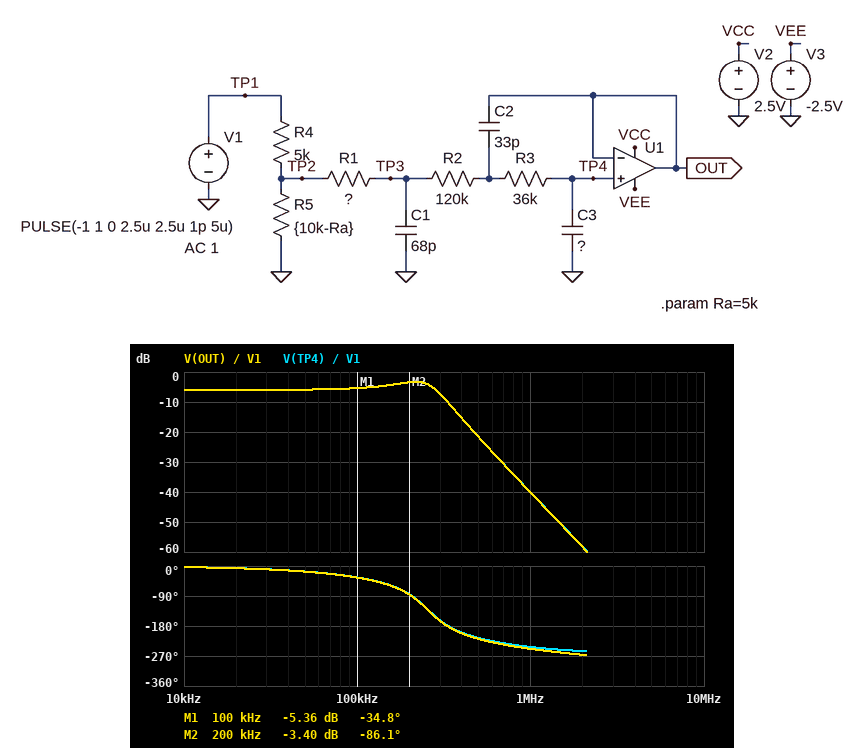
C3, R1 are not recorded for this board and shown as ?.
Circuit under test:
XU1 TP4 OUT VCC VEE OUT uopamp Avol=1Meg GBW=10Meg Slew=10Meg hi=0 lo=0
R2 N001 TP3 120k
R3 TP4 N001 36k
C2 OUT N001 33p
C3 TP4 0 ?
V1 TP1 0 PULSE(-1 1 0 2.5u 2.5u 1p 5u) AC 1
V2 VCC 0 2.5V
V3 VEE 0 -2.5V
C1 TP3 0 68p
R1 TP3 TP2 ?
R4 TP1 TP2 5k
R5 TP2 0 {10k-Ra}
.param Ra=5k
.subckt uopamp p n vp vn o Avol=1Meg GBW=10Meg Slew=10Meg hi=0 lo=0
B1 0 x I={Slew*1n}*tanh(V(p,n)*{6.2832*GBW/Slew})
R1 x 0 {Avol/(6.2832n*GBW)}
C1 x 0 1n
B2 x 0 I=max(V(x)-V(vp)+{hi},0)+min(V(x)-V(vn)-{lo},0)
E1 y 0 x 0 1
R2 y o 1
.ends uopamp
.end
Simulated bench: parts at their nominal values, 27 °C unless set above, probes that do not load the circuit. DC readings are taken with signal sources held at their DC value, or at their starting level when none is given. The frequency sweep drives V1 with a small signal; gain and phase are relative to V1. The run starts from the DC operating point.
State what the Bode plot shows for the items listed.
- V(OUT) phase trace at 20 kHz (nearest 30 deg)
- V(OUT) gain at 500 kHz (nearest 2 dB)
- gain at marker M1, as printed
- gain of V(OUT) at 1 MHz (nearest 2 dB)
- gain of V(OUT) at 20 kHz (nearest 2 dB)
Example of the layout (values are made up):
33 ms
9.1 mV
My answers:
0 deg
-22 dB
-5.36 dB
-40 dB
-6 dB
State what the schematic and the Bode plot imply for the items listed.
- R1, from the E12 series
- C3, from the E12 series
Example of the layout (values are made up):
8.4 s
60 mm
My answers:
5.6 kΩ
2.2 pF
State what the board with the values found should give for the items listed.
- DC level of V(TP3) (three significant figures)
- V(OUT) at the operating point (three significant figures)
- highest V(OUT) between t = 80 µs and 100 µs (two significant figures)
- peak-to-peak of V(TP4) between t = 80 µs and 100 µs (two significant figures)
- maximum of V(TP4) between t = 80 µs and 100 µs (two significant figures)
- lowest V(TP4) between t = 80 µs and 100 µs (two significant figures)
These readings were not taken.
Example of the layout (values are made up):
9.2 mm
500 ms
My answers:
-500 mV
-500 mV
550 mV
1.1 V
550 mV
-550 mV
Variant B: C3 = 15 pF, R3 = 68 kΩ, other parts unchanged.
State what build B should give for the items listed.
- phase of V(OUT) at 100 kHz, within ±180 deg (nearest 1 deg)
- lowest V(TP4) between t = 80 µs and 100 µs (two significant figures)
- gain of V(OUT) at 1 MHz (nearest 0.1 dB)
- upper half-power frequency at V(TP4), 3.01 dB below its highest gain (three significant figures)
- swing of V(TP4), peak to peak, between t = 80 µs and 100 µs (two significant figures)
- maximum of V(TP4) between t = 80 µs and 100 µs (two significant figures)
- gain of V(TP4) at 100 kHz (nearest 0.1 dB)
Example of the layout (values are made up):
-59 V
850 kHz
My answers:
-130 deg
-49 mV
-61.4 dB
73.4 kHz
97 mV
49 mV
-12.5 dB
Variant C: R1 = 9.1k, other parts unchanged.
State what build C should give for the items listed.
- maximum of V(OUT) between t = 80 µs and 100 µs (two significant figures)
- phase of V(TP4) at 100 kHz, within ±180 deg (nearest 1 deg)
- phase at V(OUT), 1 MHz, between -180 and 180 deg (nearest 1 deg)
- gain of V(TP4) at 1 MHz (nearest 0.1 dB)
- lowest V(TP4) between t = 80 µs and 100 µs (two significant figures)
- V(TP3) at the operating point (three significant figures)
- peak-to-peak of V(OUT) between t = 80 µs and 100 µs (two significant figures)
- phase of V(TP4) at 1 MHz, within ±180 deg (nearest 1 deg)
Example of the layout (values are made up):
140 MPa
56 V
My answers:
470 mV
-42 deg
107 deg
-43.1 dB
-470 mV
-500 mV
930 mV
112 deg
